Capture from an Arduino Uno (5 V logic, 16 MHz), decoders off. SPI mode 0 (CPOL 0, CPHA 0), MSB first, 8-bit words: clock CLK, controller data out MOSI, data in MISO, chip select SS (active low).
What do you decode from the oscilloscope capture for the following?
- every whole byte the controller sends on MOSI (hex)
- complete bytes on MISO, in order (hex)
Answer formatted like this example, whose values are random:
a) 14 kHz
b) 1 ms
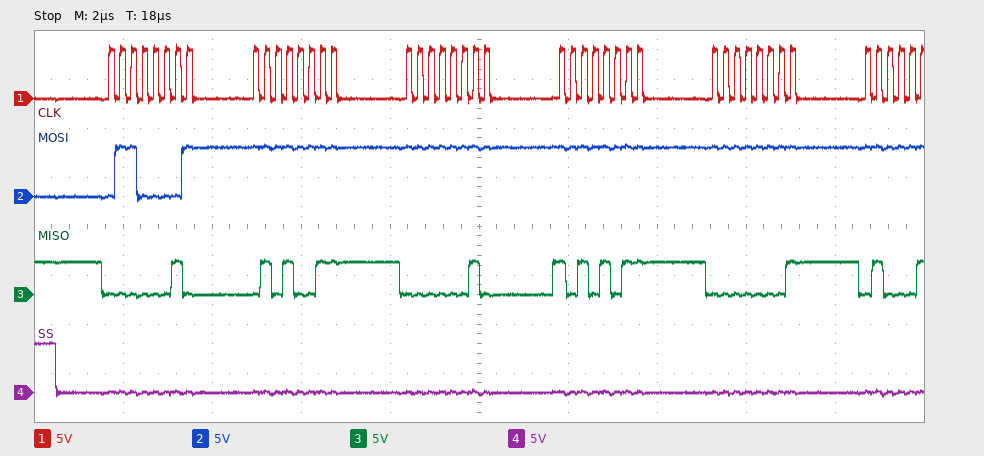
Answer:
a) 61 FF FF FF FF
b) 02 53 02 AB 01
